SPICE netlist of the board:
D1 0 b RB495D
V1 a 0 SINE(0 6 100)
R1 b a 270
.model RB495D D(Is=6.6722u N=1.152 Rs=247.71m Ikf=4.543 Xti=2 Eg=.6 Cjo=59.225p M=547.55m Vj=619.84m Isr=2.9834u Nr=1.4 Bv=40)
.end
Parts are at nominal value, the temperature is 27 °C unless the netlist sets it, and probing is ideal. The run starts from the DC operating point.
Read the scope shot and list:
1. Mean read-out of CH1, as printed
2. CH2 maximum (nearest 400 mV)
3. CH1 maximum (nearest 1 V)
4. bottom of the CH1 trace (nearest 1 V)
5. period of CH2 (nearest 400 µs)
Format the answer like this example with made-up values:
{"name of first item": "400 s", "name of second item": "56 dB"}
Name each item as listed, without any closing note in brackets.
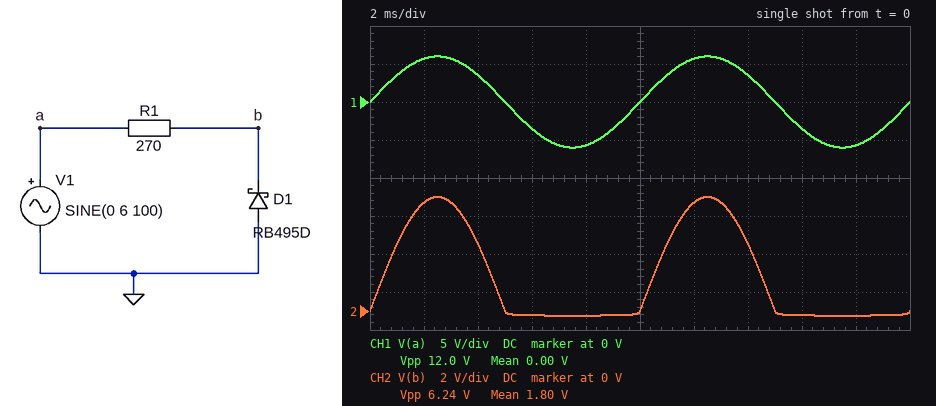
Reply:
{"Mean read-out of CH1, as printed": "0.00 V", "CH2 maximum": "6.0 V", "CH1 maximum": "6 V", "bottom of the CH1 trace": "-6 V", "period of CH2": "10.0 ms"}
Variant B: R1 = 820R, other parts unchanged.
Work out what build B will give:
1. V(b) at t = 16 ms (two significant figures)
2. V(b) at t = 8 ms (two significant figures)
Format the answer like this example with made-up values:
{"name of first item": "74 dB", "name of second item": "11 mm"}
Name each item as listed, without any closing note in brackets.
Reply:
{"V(b) at t = 16 ms": "-190 mV", "V(b) at t = 8 ms": "-210 mV"}
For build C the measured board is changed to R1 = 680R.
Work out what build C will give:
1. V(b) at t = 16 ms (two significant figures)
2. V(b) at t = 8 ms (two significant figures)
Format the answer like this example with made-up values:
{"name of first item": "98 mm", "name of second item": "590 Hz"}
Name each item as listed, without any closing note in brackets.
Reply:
{"V(b) at t = 16 ms": "-200 mV", "V(b) at t = 8 ms": "-210 mV"}
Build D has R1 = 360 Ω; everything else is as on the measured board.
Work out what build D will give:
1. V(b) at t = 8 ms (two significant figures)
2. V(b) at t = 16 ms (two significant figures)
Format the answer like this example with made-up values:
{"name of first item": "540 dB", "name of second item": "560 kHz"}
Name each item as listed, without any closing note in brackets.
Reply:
{"V(b) at t = 8 ms": "-230 mV", "V(b) at t = 16 ms": "-220 mV"}
